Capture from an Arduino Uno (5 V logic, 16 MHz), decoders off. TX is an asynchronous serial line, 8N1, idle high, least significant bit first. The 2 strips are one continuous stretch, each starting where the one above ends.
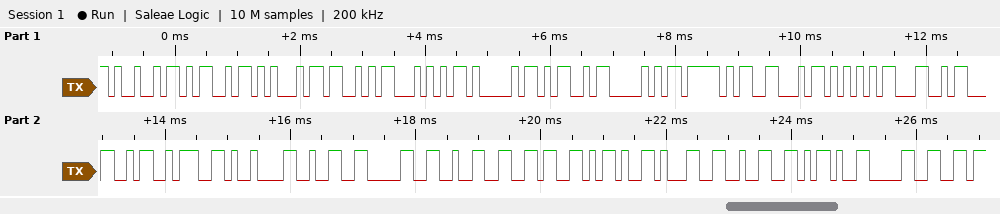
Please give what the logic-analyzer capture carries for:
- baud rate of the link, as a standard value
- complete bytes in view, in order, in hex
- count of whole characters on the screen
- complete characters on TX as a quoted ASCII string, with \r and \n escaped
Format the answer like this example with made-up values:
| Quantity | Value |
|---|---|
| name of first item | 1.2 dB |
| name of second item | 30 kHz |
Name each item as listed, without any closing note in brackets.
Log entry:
| Quantity | Value |
|---|---|
| baud rate of the link, as a standard value | 9600 baud |
| complete bytes in view, in order, in hex | 0x49 0x4D 0x45 0x53 0x54 0x41 0x4D 0x50 0x5F 0x46 0x55 0x4C 0x4C 0x3A 0x09 0x32 0x30 0x32 0x36 0x2D 0x31 0x32 0x2D 0x30 |
| count of whole characters on the screen | 24 |
| complete characters on TX as a quoted ASCII string, with \r and \n escaped | "IMESTAMP_FULL:\t2026-12-0" |
